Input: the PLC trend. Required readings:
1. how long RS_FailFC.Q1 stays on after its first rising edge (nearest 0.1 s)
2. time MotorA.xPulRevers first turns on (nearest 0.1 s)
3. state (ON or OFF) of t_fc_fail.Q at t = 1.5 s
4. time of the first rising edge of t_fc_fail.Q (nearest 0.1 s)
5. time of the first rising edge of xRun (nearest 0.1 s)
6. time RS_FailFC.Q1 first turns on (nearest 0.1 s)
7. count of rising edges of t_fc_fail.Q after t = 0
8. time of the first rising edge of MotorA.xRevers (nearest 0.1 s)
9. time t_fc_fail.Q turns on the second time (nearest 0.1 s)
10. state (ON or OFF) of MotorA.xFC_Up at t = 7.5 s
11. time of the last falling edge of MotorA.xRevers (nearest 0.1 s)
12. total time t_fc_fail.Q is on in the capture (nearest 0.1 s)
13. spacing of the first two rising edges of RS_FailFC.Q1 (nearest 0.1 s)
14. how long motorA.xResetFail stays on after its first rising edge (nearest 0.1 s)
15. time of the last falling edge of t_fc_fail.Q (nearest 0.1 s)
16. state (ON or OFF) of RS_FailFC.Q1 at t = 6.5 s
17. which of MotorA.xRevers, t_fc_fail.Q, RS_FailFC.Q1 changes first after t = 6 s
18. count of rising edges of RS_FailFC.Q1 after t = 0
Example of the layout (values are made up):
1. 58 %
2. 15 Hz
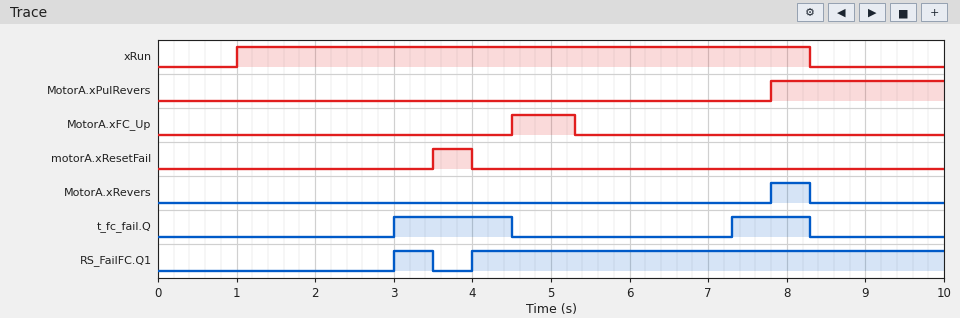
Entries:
1. 0.5 s
2. 7.8 s
3. OFF
4. 3.0 s
5. 1.0 s
6. 3.0 s
7. 2
8. 7.8 s
9. 7.3 s
10. OFF
11. 8.3 s
12. 2.5 s
13. 1.0 s
14. 0.5 s
15. 8.3 s
16. ON
17. t_fc_fail.Q
18. 2
